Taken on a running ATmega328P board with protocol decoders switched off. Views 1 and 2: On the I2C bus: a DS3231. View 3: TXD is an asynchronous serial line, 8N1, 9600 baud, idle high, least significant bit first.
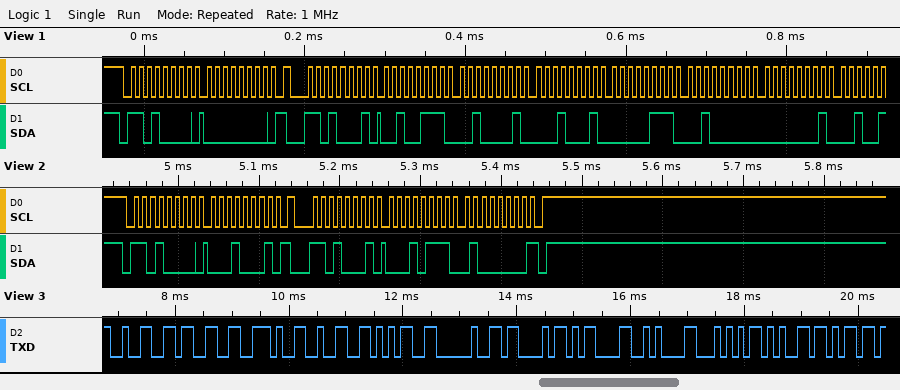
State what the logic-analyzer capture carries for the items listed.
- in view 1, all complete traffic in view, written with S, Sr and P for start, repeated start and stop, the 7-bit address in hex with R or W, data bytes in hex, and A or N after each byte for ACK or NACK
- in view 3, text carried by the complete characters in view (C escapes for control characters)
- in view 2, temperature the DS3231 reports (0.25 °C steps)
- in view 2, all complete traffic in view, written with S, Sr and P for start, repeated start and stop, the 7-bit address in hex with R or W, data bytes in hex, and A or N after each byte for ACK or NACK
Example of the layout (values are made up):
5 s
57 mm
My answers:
S 68W A 00 A Sr 68R A 27 A 21 A 11 A 07 A 20 A 01 A
"23.25 C\r\nTem"
23.25 °C
S 68W A 11 A Sr 68R A 17 A 40 N P
